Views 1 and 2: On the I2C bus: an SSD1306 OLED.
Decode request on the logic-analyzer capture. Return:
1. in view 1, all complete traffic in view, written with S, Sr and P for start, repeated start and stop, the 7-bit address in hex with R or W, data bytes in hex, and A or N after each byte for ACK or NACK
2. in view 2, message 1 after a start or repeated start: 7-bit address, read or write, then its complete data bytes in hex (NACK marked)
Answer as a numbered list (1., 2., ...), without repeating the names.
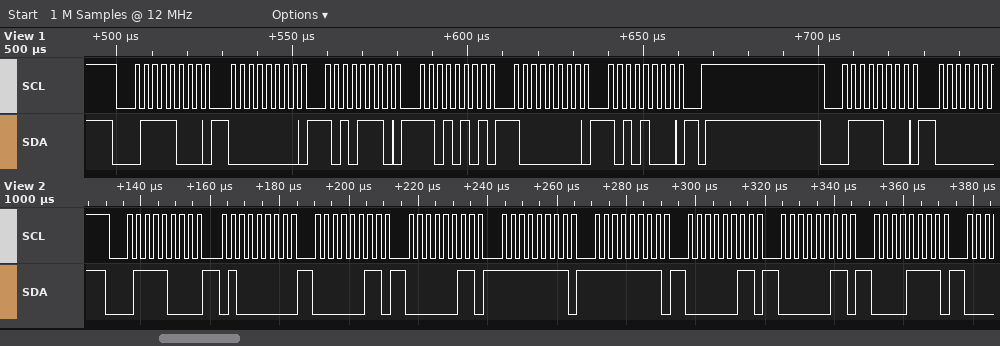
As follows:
1. S 3CW A 00 A AE A D5 A 80 A A8 A P S 3CW A
2. 0x3C write: 40 03 03 FF FF 03 03 0F
